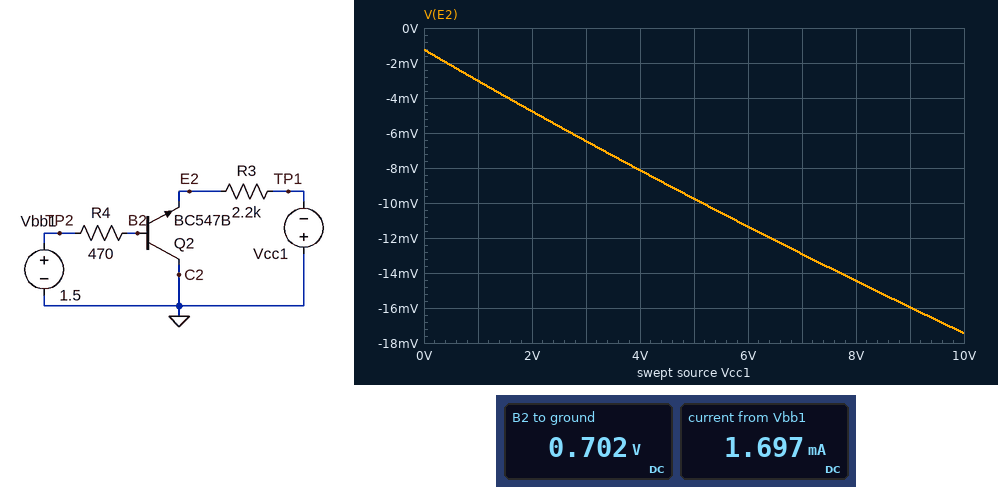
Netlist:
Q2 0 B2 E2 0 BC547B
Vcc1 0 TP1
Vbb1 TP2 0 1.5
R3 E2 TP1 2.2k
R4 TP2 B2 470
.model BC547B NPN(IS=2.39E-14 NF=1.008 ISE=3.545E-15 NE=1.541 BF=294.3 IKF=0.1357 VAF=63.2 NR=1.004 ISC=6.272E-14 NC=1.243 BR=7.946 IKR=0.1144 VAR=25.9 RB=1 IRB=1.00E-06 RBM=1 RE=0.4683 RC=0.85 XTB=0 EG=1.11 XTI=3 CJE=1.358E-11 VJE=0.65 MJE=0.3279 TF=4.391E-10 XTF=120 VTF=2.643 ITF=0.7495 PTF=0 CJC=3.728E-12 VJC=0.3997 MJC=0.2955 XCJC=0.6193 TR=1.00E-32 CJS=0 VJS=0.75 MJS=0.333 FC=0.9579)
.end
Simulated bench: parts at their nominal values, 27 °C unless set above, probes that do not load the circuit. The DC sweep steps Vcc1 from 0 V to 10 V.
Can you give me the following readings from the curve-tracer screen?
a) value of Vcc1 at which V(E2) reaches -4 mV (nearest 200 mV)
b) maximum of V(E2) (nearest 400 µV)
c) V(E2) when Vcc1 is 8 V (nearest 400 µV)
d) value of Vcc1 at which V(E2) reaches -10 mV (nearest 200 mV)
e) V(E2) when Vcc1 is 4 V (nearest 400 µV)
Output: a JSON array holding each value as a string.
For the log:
["1.6 V", "-1.2 mV", "-14.4 mV", "5.2 V", "-8.0 mV"]
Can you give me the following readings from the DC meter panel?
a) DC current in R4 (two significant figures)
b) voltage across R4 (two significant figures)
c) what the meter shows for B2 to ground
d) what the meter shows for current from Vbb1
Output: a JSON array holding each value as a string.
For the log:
["1.7 mA", "800 mV", "0.702 V", "1.697 mA"]
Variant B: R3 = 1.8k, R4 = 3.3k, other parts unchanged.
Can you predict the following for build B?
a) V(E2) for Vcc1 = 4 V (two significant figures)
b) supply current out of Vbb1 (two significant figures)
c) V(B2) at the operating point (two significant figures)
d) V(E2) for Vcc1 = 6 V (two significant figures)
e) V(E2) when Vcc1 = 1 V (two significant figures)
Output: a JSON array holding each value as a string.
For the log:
["-28 mV", "260 µA", "650 mV", "-37 mV", "-11 mV"]
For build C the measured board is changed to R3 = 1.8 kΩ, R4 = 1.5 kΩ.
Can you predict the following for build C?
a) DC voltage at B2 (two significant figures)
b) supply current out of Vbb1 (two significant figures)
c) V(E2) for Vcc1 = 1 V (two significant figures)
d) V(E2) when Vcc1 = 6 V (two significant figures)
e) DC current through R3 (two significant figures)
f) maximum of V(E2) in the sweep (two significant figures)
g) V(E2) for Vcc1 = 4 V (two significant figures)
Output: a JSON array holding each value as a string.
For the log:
["670 mV", "550 µA", "-6.8 mV", "-25 mV", "1.2 µA", "-2.1 mV", "-18 mV"]
